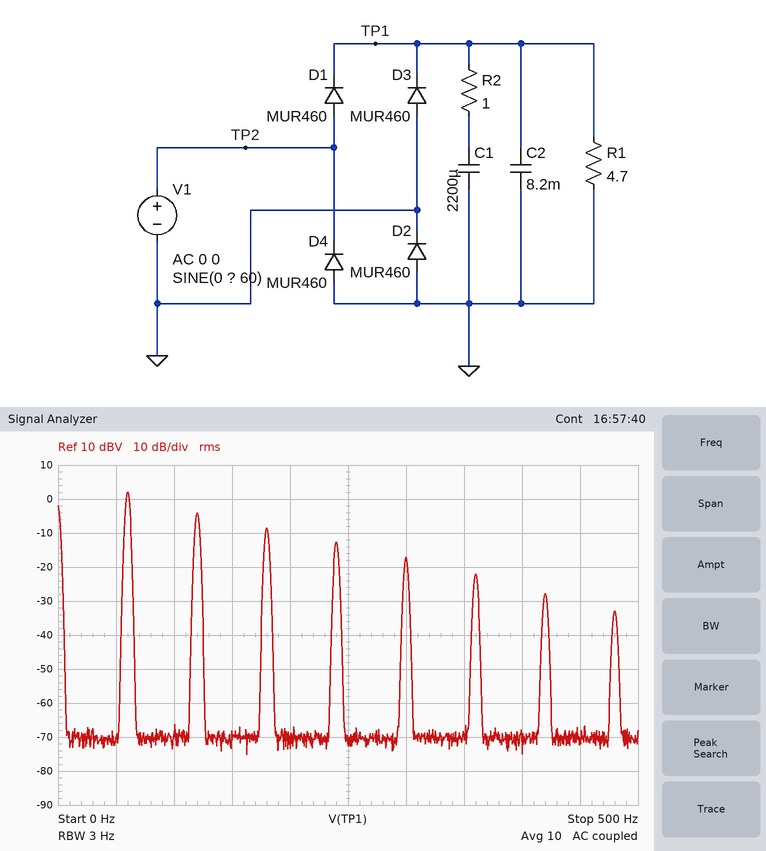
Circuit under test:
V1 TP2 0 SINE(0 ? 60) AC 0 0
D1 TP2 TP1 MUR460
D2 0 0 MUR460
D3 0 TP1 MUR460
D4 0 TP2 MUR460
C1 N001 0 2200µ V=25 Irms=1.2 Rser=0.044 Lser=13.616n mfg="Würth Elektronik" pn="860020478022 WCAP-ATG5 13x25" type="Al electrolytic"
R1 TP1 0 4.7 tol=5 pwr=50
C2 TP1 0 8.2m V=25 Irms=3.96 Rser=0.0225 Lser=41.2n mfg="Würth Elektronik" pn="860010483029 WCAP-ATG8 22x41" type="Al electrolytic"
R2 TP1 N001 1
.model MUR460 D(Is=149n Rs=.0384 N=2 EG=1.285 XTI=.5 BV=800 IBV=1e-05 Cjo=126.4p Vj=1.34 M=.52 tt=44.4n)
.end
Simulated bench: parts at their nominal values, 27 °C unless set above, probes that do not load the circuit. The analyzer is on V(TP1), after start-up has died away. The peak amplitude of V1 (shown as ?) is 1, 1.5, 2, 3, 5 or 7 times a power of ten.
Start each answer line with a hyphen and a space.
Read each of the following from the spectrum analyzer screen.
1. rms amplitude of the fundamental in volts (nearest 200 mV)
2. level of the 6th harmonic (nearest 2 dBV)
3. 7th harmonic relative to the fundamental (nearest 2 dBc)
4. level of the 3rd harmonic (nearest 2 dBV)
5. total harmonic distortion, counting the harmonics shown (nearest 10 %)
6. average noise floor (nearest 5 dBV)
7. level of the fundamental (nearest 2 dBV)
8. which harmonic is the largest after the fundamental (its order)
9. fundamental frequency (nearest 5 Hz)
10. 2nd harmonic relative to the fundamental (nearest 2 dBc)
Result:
- 1.2 V
- -22 dBV
- -30 dBc
- -8 dBV
- 60 %
- -70 dBV
- 2 dBV
- 2
- 60 Hz
- -6 dBc
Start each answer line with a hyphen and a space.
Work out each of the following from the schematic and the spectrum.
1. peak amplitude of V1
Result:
- 20 V
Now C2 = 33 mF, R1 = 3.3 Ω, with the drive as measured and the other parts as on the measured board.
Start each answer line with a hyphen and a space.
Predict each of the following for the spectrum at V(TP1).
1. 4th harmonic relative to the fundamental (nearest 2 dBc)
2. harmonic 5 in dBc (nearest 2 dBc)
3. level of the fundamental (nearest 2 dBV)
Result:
- -12 dBc
- -16 dBc
- -6 dBV
